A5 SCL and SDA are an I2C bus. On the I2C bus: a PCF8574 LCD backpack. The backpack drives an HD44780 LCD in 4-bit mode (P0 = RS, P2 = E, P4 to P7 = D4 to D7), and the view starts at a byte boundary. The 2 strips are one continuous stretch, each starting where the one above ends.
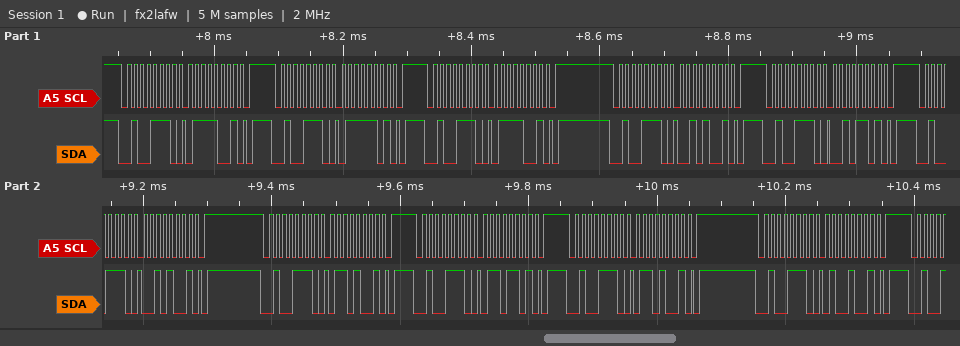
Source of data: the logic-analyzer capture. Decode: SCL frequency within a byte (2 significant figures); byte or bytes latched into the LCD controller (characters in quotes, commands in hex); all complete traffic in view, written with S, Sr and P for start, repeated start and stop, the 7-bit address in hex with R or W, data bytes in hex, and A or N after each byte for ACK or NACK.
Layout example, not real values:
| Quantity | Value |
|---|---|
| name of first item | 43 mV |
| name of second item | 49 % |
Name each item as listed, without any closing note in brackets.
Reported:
| Quantity | Value |
|---|---|
| SCL frequency within a byte | 100 kHz |
| byte or bytes latched into the LCD controller | 'r' |
| all complete traffic in view, written with S, Sr and P for start, repeated start and stop, the 7-bit address in hex with R or W, data bytes in hex, and A or N after each byte for ACK or NACK | S 27W A 79 A P S 27W A 7D A P S 27W A 79 A P S 27W A 29 A P S 27W A 2D A P S 27W A 29 A P S 27W A 69 A P S 27W A 6D A P S 27W A 69 A P S 27W A 49 A P |
